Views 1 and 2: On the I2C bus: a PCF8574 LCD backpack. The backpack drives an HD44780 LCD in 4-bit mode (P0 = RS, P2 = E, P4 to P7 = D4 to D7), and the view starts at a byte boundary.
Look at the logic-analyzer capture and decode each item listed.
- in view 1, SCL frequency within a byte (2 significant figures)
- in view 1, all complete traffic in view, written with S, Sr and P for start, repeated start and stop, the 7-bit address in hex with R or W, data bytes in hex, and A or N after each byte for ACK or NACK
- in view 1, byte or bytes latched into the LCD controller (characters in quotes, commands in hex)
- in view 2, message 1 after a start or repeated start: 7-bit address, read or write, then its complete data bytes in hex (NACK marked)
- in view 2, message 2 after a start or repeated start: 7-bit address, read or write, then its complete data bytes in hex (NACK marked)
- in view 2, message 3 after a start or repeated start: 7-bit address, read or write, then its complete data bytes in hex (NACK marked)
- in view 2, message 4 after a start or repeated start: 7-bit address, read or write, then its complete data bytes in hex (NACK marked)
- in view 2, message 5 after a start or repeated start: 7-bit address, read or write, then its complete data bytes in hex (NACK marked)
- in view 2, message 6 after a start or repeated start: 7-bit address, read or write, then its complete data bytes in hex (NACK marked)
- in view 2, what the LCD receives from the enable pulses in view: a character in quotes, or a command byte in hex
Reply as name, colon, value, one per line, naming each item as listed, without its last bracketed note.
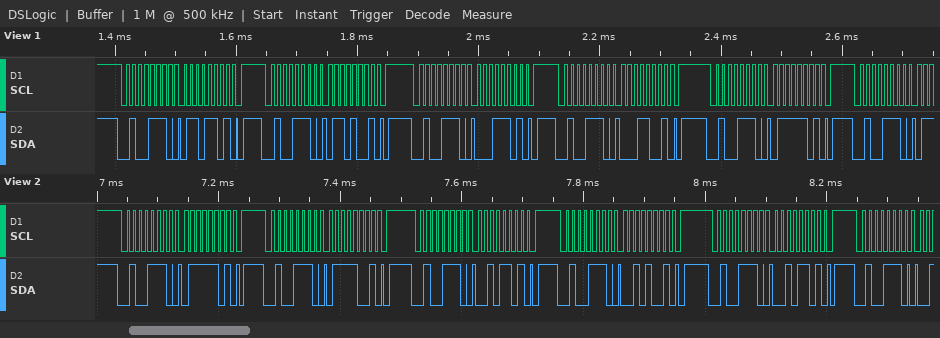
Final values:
in view 1, SCL frequency within a byte: 100 kHz
in view 1, all complete traffic in view, written with S, Sr and P for start, repeated start and stop, the 7-bit address in hex with R or W, data bytes in hex, and A or N after each byte for ACK or NACK: S 27W A 6D A P S 27W A 69 A P S 27W A 1D A P S 27W A 19 A P S 27W A 7D A P S 27W A
in view 1, byte or bytes latched into the LCD controller: 'a'
in view 2, message 1 after a start or repeated start: 7-bit address, read or write, then its complete data bytes in hex: 0x27 write: 7D
in view 2, message 2 after a start or repeated start: 7-bit address, read or write, then its complete data bytes in hex: 0x27 write: 79
in view 2, message 3 after a start or repeated start: 7-bit address, read or write, then its complete data bytes in hex: 0x27 write: 2D
in view 2, message 4 after a start or repeated start: 7-bit address, read or write, then its complete data bytes in hex: 0x27 write: 29
in view 2, message 5 after a start or repeated start: 7-bit address, read or write, then its complete data bytes in hex: 0x27 write: 2D
in view 2, message 6 after a start or repeated start: 7-bit address, read or write, then its complete data bytes in hex: 0x27 write
in view 2, what the LCD receives from the enable pulses in view: a character in quotes, or a command byte in hex: 'r'
